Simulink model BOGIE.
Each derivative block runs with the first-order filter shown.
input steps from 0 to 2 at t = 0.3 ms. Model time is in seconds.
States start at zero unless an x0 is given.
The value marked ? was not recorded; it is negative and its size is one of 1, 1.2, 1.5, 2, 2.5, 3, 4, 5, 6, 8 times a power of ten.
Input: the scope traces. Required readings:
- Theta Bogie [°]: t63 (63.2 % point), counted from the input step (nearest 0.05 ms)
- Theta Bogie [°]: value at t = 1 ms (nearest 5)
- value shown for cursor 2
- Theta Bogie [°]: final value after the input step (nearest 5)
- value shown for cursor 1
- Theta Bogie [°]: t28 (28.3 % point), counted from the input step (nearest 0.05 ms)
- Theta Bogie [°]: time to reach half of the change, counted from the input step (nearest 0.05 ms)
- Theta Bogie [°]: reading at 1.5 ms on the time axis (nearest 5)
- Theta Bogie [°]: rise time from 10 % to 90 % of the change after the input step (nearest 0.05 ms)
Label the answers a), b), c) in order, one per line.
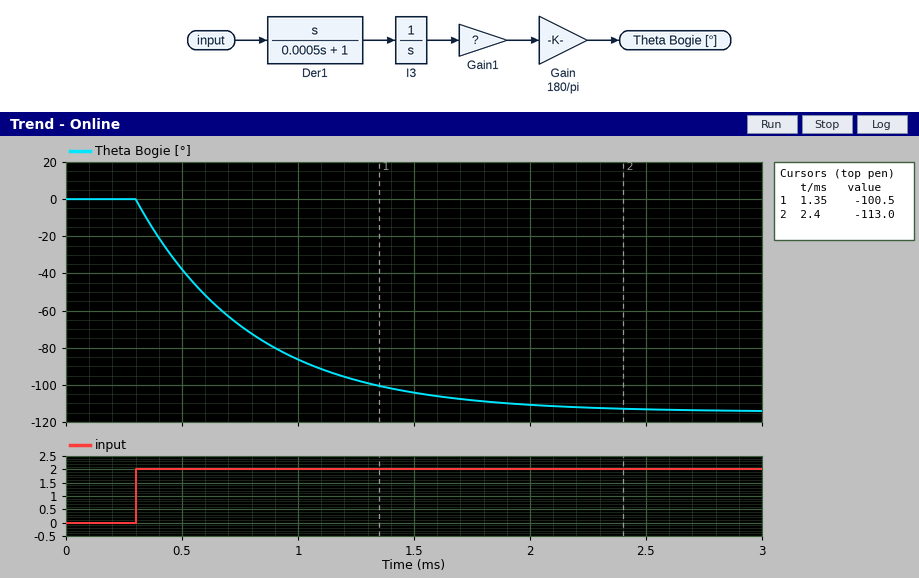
a) 0.50 ms
b) -85
c) -113.0
d) -115
e) -100.5
f) 0.15 ms
g) 0.35 ms
h) -105
i) 1.10 ms
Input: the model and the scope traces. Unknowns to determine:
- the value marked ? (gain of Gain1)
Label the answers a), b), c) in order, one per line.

a) -1
